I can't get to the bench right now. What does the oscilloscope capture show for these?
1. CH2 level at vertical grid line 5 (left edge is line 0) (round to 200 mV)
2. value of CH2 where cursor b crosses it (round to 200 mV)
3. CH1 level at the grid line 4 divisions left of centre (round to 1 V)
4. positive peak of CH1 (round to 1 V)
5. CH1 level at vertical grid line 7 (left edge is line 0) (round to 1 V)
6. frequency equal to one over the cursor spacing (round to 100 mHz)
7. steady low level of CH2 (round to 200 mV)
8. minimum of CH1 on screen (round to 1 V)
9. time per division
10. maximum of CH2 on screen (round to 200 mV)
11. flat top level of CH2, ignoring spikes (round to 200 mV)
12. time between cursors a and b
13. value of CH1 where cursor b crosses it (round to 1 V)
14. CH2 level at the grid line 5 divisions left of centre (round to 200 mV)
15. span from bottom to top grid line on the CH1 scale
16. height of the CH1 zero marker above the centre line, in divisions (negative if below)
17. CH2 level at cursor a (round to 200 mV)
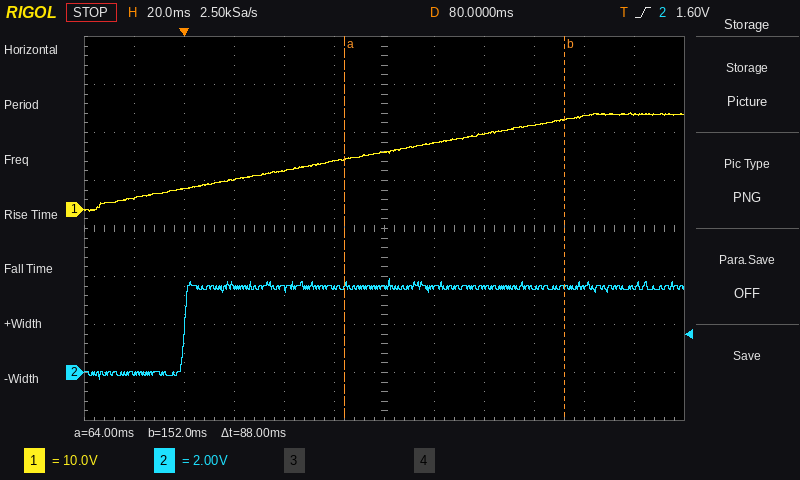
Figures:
3.6 V
3.6 V
4 V
20 V
14 V
11.4 Hz
0.0 V
0 V
20 ms
4.0 V
3.6 V
88 ms
19 V
0.0 V
80 V
+0.4 div
3.6 V
